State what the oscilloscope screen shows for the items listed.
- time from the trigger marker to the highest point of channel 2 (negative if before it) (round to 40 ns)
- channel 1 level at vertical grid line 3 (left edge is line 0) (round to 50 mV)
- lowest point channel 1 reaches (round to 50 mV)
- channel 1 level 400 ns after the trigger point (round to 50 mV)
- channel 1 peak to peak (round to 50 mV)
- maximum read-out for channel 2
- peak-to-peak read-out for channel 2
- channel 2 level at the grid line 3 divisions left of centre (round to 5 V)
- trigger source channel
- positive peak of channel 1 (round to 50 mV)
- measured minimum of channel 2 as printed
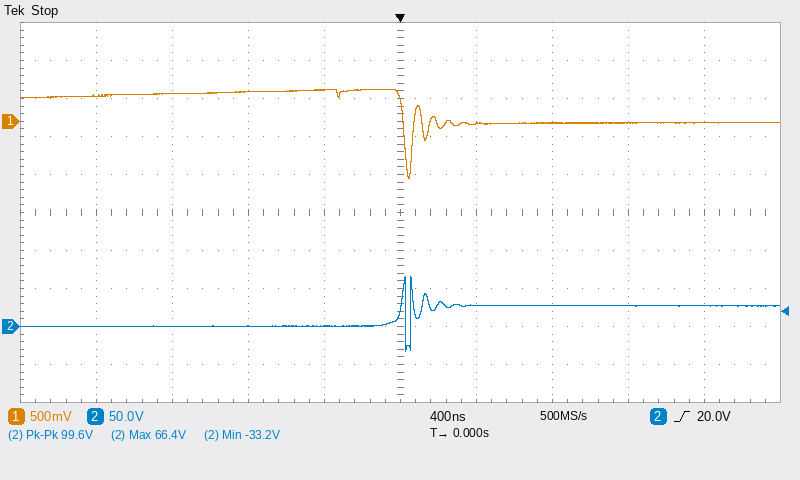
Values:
+40 ns
400 mV
-750 mV
-50 mV
1.15 V
66.4 V
99.6 V
0 V
channel 2
400 mV
-33.2 V
